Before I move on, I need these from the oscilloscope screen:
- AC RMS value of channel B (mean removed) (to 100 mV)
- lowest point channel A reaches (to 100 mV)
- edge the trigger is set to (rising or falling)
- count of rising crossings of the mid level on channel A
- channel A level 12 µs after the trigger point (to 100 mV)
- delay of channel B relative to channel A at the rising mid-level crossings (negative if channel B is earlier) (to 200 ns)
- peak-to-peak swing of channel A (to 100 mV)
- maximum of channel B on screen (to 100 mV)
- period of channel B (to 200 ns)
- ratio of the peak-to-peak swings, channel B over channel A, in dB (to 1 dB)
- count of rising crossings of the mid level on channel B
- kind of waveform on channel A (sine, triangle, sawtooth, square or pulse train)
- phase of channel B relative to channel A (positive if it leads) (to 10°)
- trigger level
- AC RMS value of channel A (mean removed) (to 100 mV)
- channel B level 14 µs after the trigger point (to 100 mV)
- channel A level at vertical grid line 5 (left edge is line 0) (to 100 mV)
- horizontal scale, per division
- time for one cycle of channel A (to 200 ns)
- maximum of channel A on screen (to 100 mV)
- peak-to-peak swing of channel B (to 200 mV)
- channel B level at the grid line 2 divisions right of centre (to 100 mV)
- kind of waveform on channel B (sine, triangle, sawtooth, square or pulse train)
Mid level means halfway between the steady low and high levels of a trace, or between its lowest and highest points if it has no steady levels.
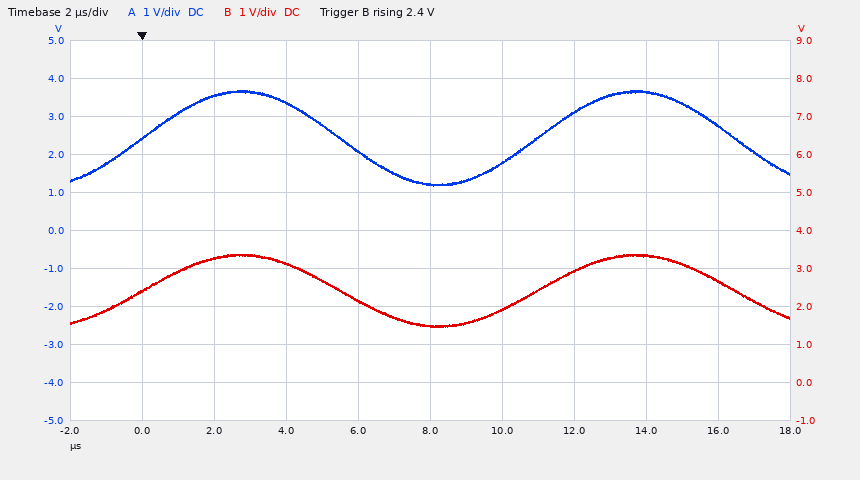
700 mV
1.2 V
rising
2
3.1 V
0.0 µs
2.5 V
3.4 V
11.0 µs
-2 dB
2
sine
0°
2.4 V
900 mV
3.3 V
1.2 V
2 µs
11.0 µs
3.7 V
2.0 V
2.9 V
sine
